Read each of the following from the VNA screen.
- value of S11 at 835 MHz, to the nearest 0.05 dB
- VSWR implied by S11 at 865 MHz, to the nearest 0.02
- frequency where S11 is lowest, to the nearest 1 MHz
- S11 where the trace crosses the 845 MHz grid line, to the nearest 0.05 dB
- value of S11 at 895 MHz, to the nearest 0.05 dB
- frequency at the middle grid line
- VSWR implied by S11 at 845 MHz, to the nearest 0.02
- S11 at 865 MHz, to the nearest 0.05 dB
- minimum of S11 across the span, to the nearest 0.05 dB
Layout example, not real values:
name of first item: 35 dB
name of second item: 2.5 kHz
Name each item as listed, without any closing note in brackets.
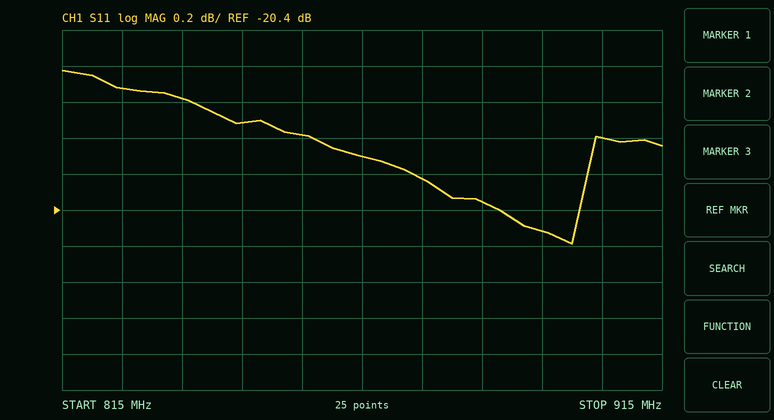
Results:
value of S11 at 835 MHz, to the nearest 0.05 dB: -19.80 dB
VSWR implied by S11 at 865 MHz, to the nearest 0.02: 1.22
frequency where S11 is lowest, to the nearest 1 MHz: 900 MHz
S11 where the trace crosses the 845 MHz grid line, to the nearest 0.05 dB: -19.90 dB
value of S11 at 895 MHz, to the nearest 0.05 dB: -20.50 dB
frequency at the middle grid line: 865 MHz
VSWR implied by S11 at 845 MHz, to the nearest 0.02: 1.22
S11 at 865 MHz, to the nearest 0.05 dB: -20.10 dB
minimum of S11 across the span, to the nearest 0.05 dB: -20.60 dB
